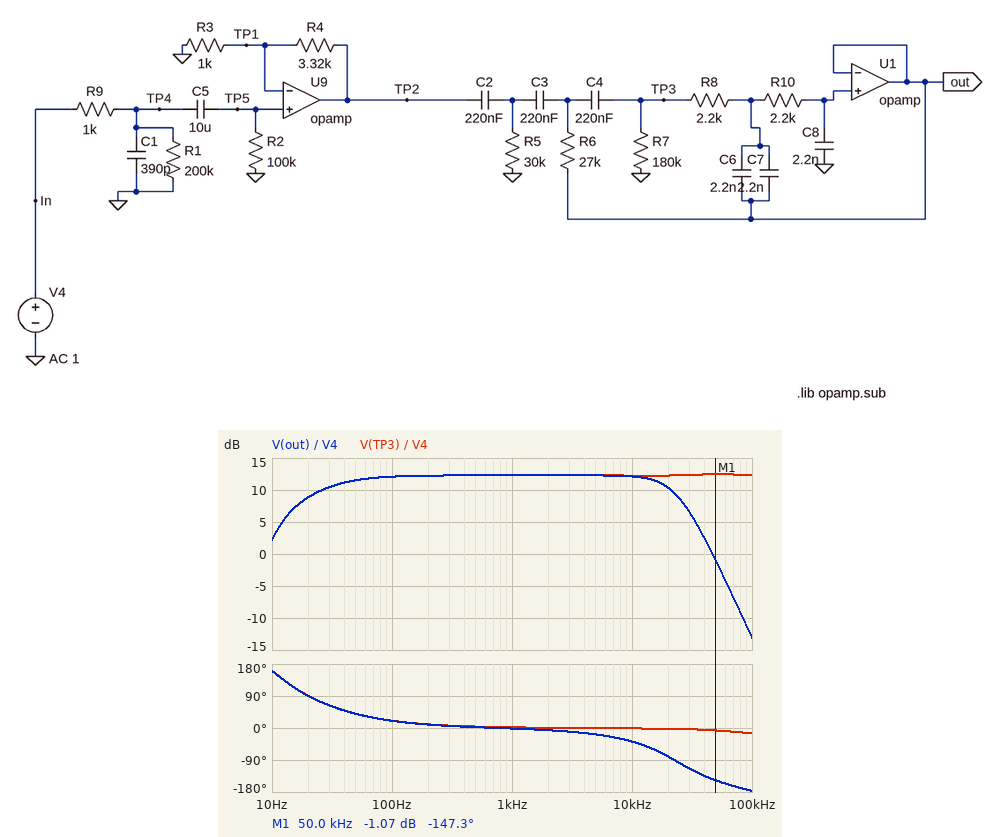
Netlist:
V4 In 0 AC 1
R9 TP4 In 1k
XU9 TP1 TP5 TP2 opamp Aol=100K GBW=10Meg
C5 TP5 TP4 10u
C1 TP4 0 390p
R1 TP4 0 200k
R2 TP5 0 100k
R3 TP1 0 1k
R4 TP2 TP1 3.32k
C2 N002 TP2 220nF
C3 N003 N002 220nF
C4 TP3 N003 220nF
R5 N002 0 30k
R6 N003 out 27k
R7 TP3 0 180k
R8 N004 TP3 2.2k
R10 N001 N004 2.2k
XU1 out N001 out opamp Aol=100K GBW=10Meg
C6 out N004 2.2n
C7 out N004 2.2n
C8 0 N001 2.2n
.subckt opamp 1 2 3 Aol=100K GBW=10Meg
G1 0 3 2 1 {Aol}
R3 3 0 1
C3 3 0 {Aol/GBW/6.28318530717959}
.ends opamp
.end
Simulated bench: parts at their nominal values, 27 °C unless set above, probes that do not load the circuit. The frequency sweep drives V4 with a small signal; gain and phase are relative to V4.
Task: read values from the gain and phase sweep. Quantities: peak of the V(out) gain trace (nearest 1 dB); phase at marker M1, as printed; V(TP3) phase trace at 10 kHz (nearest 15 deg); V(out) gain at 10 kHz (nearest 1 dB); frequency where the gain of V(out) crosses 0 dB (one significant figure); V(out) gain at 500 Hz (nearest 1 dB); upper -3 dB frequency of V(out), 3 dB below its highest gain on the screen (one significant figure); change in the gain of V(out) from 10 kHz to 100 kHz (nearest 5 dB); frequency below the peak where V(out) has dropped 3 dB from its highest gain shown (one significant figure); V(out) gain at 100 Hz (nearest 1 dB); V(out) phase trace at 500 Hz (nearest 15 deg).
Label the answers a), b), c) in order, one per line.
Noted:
a) 12 dB
b) -147.3 deg
c) 0 deg
d) 12 dB
e) 50 kHz
f) 12 dB
g) 20 kHz
h) -25 dB
i) 20 Hz
j) 12 dB
k) 0 deg
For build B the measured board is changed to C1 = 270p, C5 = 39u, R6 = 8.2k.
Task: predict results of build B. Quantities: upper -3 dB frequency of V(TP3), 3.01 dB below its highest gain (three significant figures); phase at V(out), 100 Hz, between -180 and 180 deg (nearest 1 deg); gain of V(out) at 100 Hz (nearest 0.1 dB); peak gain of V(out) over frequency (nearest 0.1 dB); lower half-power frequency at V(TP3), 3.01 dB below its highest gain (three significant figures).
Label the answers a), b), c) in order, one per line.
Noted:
a) 504 kHz
b) 21 deg
c) 12.4 dB
d) 13.1 dB
e) 21.5 Hz
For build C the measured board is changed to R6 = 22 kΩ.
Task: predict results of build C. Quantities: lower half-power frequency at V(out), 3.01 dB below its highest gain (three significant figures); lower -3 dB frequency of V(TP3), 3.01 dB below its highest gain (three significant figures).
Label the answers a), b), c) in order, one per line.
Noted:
a) 20.3 Hz
b) 21.0 Hz
